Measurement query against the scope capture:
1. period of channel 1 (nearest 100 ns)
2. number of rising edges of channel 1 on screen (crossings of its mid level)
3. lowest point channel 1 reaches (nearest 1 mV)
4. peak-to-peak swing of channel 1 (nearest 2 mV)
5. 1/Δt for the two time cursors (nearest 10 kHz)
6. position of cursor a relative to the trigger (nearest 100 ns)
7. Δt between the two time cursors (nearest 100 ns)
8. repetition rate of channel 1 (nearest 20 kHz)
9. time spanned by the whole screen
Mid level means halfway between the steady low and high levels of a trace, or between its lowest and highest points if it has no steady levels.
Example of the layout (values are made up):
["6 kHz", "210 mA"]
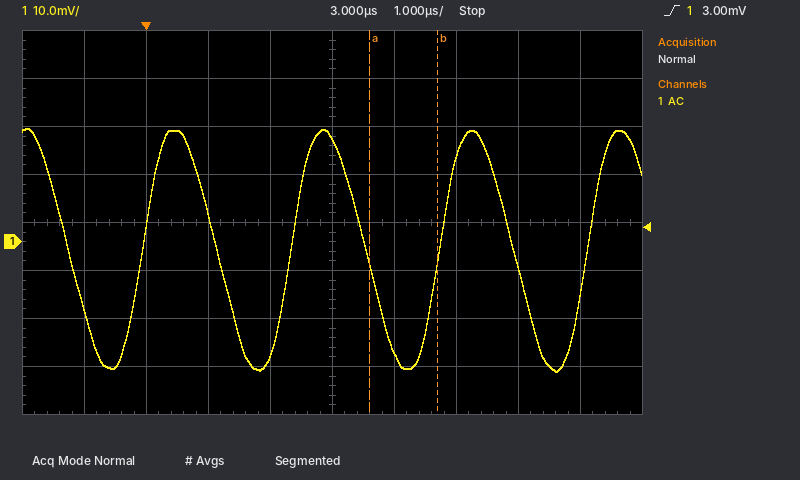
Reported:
["2.4 µs", "4", "-27 mV", "50 mV", "910 kHz", "+3.6 µs", "1.1 µs", "420 kHz", "10 µs"]
